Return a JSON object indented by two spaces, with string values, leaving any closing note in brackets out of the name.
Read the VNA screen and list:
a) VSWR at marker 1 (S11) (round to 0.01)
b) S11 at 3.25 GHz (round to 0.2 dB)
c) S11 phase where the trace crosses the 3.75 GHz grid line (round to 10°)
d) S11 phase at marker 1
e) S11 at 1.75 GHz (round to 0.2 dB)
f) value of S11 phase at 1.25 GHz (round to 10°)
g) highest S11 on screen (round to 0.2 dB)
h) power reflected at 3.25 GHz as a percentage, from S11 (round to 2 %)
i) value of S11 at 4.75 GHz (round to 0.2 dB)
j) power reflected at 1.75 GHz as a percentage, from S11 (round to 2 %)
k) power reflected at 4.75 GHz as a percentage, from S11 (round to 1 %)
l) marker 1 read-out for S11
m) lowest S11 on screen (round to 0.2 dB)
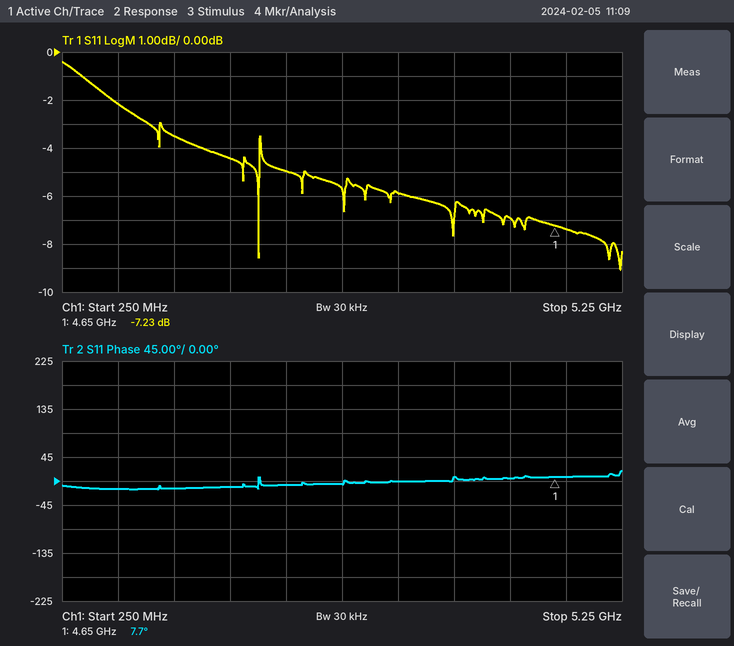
{
  "VSWR at marker 1 (S11)": "2.54",
  "S11 at 3.25 GHz": "-5.8 dB",
  "S11 phase where the trace crosses the 3.75 GHz grid line": "10°",
  "S11 phase at marker 1": "7.7°",
  "S11 at 1.75 GHz": "-4.4 dB",
  "value of S11 phase at 1.25 GHz": "-10°",
  "highest S11 on screen": "-0.4 dB",
  "power reflected at 3.25 GHz as a percentage, from S11": "26 %",
  "value of S11 at 4.75 GHz": "-7.4 dB",
  "power reflected at 1.75 GHz as a percentage, from S11": "36 %",
  "power reflected at 4.75 GHz as a percentage, from S11": "18 %",
  "marker 1 read-out for S11": "-7.23 dB",
  "lowest S11 on screen": "-9.0 dB"
}
